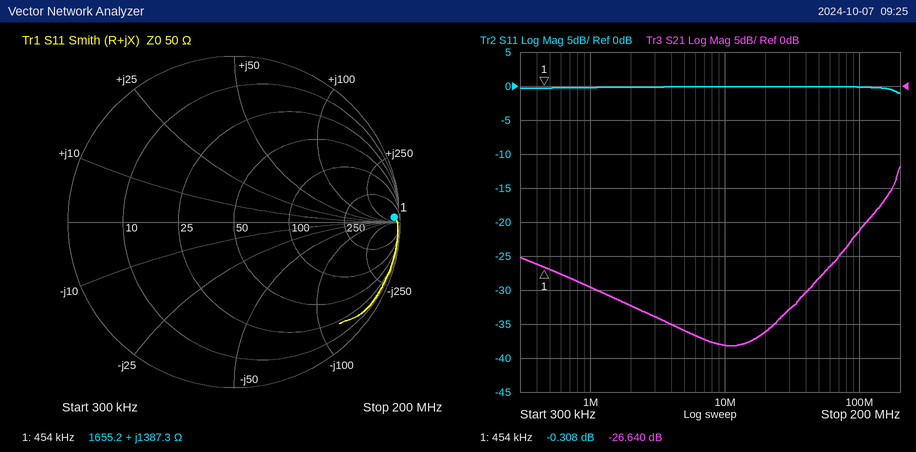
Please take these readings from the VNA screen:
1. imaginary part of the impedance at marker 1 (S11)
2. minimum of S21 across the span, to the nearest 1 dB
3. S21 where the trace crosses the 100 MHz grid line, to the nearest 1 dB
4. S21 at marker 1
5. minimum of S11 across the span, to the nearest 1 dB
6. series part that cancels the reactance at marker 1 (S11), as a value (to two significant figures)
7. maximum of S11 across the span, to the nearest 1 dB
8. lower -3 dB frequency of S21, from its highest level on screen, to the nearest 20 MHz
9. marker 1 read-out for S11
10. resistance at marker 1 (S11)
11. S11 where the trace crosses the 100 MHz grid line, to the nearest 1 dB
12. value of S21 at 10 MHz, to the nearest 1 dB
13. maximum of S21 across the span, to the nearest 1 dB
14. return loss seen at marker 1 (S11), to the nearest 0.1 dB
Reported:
+1387.3 Ω
-38 dB
-21 dB
-26.640 dB
-1 dB
250 pF
0 dB
180 MHz
-0.308 dB
1655.2 Ω
0 dB
-38 dB
-12 dB
0.3 dB
